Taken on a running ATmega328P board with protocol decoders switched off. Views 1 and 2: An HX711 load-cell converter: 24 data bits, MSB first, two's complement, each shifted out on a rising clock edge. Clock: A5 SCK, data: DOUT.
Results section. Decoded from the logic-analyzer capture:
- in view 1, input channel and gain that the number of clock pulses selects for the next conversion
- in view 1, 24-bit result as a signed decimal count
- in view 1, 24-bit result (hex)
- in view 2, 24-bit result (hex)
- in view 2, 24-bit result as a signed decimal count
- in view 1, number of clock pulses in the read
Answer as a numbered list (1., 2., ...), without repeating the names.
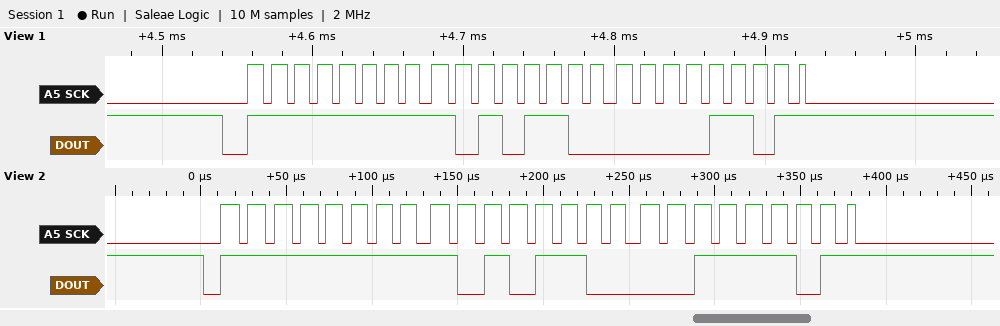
1. channel A, gain 128
2. -21491
3. 0xFFAC0D
4. 0xFFAC3D
5. -21443
6. 25
